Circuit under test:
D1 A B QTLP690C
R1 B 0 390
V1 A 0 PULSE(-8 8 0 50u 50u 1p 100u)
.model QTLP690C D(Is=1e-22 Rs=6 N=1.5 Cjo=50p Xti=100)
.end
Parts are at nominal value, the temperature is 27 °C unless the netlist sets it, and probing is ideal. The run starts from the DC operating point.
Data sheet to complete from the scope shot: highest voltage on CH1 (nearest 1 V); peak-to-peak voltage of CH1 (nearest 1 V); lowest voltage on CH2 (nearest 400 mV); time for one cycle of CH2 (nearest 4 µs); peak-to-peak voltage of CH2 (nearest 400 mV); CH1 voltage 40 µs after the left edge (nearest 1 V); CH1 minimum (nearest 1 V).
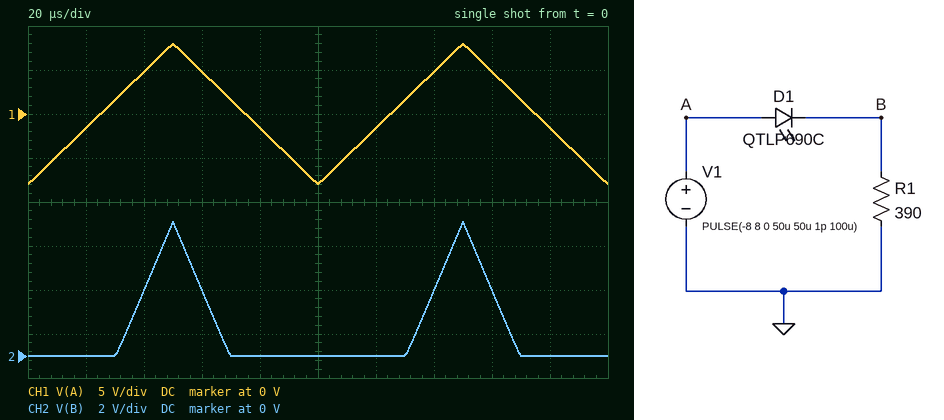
8 V
16 V
0 V
100 µs
6.0 V
5 V
-8 V
